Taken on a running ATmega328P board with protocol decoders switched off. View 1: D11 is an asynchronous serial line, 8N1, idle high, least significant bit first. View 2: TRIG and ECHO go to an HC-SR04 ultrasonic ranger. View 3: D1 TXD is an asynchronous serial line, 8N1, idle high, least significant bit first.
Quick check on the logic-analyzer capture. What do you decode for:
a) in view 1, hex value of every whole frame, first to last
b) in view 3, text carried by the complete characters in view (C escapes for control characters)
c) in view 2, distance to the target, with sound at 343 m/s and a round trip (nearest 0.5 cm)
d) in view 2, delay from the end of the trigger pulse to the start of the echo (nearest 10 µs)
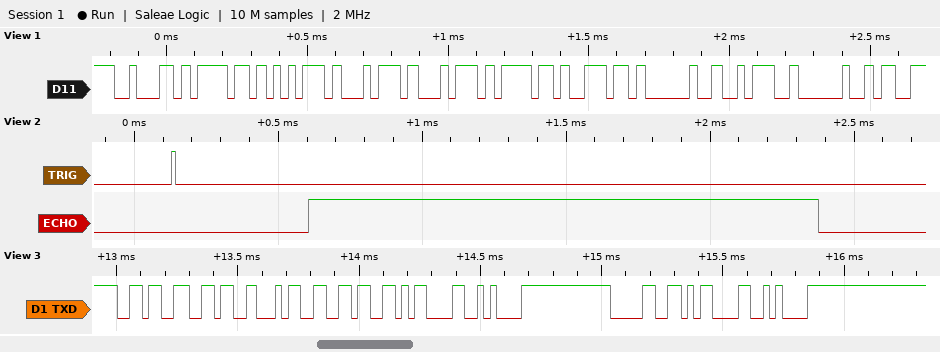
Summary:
62 6F 75 74 74 6F 6E 20 3A 20
"6646\r\n0\r\n"
30.5 cm
460 µs
